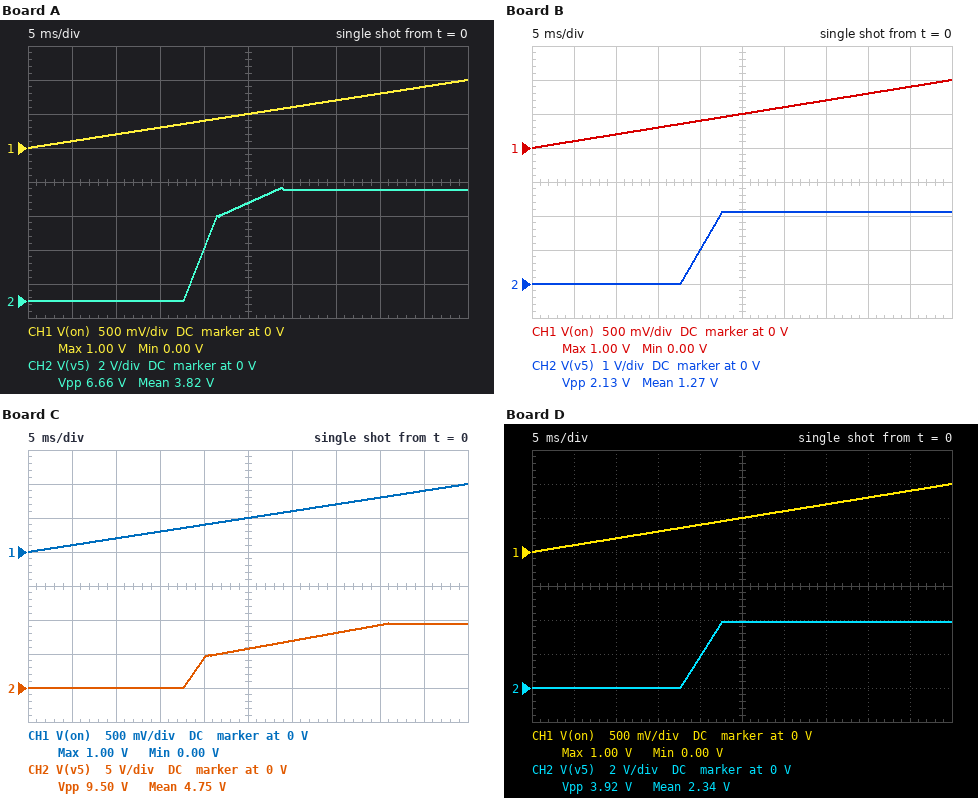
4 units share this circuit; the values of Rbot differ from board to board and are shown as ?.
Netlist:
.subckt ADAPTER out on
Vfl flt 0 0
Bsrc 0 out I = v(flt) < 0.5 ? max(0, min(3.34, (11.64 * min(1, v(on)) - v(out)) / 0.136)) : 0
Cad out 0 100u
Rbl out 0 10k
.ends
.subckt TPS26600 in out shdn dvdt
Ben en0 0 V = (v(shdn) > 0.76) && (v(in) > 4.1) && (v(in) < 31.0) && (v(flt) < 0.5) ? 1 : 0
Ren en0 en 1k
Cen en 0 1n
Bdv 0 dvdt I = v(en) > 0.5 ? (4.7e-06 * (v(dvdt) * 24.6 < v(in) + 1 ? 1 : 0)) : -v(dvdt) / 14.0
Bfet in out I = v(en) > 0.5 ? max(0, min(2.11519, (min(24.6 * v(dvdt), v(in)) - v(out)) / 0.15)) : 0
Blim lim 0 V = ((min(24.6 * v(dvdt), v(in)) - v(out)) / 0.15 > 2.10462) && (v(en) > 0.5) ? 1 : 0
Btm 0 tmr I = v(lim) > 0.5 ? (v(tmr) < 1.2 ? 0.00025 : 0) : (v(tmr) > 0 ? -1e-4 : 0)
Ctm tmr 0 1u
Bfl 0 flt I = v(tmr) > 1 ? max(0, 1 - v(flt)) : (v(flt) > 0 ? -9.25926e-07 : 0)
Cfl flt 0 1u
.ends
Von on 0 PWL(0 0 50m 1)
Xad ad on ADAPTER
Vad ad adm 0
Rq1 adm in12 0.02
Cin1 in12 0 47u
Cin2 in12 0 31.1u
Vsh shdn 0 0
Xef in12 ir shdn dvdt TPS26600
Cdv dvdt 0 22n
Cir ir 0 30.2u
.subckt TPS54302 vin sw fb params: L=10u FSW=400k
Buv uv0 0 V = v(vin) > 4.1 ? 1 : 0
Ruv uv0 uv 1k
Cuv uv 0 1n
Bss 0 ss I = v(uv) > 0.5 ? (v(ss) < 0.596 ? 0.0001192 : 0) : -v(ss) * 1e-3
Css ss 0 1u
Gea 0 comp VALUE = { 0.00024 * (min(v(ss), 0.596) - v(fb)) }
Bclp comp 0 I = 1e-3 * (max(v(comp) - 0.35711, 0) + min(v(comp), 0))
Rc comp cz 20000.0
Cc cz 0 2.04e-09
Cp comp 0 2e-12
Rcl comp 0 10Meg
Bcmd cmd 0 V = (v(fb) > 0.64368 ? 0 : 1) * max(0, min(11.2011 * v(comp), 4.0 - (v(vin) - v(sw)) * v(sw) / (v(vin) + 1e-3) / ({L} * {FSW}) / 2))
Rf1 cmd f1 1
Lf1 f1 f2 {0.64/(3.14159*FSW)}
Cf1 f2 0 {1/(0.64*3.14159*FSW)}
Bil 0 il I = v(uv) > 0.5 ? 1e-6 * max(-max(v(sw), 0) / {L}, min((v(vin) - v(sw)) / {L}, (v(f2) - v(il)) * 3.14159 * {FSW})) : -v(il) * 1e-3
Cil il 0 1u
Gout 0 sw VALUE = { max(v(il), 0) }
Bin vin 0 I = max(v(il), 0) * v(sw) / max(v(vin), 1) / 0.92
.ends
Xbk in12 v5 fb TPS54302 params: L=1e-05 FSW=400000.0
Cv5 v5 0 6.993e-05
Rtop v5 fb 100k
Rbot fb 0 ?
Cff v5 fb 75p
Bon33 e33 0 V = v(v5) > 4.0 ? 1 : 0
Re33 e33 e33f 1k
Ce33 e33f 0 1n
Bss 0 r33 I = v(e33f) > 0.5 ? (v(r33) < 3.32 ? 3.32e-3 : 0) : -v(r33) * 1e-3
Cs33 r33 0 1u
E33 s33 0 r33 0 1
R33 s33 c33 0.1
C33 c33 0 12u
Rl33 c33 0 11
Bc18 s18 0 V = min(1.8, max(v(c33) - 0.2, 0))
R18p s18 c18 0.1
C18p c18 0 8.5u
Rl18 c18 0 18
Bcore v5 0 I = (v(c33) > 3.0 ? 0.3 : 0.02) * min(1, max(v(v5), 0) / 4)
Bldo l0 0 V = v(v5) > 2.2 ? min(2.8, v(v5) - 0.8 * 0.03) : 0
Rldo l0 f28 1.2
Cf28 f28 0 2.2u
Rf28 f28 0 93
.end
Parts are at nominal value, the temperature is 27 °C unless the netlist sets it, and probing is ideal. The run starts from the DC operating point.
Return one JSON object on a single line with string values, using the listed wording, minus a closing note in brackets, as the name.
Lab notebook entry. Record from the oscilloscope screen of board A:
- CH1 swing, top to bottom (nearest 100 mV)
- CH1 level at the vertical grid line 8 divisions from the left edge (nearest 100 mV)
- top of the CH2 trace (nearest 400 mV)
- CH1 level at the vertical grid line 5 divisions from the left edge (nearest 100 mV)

{"CH1 swing, top to bottom": "1.0 V", "CH1 level at the vertical grid line 8 divisions from the left edge": "800 mV", "top of the CH2 trace": "6.8 V", "CH1 level at the vertical grid line 5 divisions from the left edge": "500 mV"}
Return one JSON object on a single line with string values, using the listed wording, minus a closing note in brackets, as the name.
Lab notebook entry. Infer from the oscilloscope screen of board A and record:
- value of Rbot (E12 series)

{"value of Rbot": "10 kΩ"}
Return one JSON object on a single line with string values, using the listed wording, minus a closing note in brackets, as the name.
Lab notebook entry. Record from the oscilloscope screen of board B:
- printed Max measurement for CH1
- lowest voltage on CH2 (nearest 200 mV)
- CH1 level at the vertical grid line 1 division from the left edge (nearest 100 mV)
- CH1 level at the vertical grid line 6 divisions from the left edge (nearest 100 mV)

{"printed Max measurement for CH1": "1.00 V", "lowest voltage on CH2": "0 V", "CH1 level at the vertical grid line 1 division from the left edge": "100 mV", "CH1 level at the vertical grid line 6 divisions from the left edge": "600 mV"}
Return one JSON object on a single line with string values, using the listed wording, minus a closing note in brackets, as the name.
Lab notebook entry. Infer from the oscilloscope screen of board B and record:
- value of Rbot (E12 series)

{"value of Rbot": "39 kΩ"}
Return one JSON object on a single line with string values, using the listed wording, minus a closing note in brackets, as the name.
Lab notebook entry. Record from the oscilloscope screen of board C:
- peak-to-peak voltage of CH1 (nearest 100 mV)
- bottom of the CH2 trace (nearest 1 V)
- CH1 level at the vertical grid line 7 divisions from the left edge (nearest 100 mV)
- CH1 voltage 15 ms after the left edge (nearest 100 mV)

{"peak-to-peak voltage of CH1": "1.0 V", "bottom of the CH2 trace": "0 V", "CH1 level at the vertical grid line 7 divisions from the left edge": "700 mV", "CH1 voltage 15 ms after the left edge": "300 mV"}
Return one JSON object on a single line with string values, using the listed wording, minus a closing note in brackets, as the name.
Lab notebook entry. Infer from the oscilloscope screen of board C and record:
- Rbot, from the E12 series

{"Rbot, from the E12 series": "6.8 kΩ"}
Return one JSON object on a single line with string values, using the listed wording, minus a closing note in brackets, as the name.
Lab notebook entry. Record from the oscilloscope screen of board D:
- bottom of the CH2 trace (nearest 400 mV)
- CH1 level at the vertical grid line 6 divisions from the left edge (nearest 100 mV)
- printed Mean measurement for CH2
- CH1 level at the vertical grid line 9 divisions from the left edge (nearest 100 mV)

{"bottom of the CH2 trace": "0 V", "CH1 level at the vertical grid line 6 divisions from the left edge": "600 mV", "printed Mean measurement for CH2": "2.34 V", "CH1 level at the vertical grid line 9 divisions from the left edge": "900 mV"}
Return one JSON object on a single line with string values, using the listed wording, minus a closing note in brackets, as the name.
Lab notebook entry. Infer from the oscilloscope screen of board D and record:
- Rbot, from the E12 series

{"Rbot, from the E12 series": "18 kΩ"}
